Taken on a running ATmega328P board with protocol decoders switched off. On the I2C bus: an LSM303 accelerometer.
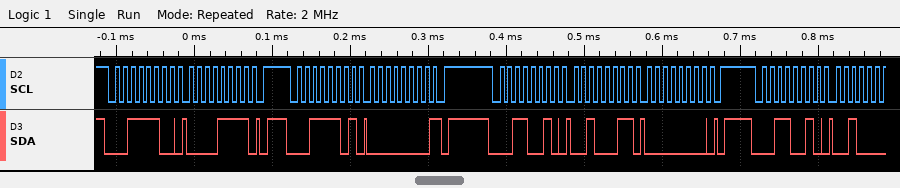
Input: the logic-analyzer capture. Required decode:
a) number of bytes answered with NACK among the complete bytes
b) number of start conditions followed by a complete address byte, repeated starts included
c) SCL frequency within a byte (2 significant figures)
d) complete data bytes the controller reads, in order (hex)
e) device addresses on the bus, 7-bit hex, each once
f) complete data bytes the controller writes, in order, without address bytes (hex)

1
4
100 kHz
00
0x1E 0x19
0F 23 00
